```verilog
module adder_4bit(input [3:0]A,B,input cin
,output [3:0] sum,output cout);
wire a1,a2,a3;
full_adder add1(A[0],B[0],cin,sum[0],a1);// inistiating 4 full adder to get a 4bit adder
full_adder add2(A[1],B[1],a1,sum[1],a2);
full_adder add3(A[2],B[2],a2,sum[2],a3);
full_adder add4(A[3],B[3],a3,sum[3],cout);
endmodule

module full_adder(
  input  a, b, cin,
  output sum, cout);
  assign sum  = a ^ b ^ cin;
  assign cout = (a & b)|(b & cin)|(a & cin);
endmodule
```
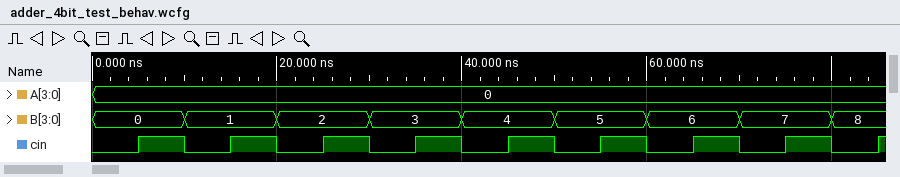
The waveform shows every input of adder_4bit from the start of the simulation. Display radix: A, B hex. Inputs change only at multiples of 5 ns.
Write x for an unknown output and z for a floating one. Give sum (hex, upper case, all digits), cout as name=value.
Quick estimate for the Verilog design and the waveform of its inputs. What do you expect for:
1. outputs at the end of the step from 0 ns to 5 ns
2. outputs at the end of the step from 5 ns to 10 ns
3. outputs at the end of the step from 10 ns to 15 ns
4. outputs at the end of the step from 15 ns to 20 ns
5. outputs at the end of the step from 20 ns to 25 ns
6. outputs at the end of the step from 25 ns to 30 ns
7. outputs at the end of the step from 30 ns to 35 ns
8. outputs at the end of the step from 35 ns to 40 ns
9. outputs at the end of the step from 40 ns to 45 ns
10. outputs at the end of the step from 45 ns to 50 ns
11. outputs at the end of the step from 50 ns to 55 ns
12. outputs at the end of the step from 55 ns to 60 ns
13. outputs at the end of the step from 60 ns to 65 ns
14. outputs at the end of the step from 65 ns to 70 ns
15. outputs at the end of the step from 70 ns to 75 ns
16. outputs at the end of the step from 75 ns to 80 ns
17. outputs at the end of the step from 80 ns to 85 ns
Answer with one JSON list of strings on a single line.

["sum=0, cout=0", "sum=1, cout=0", "sum=1, cout=0", "sum=2, cout=0", "sum=2, cout=0", "sum=3, cout=0", "sum=3, cout=0", "sum=4, cout=0", "sum=4, cout=0", "sum=5, cout=0", "sum=5, cout=0", "sum=6, cout=0", "sum=6, cout=0", "sum=7, cout=0", "sum=7, cout=0", "sum=8, cout=0", "sum=8, cout=0"]
